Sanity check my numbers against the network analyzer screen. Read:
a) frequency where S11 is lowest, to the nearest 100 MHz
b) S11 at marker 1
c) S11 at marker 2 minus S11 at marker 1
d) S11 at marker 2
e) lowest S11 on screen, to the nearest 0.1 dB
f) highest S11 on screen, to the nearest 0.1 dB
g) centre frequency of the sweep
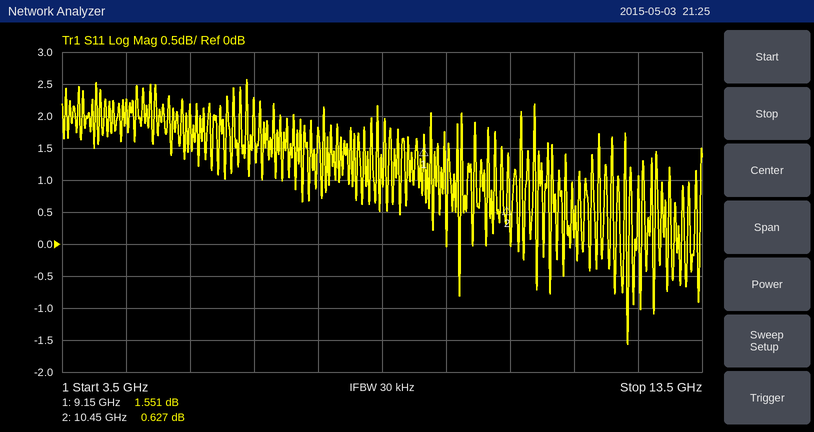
12.3 GHz
1.551 dB
-0.924 dB
0.627 dB
-1.6 dB
2.6 dB
8.5 GHz
